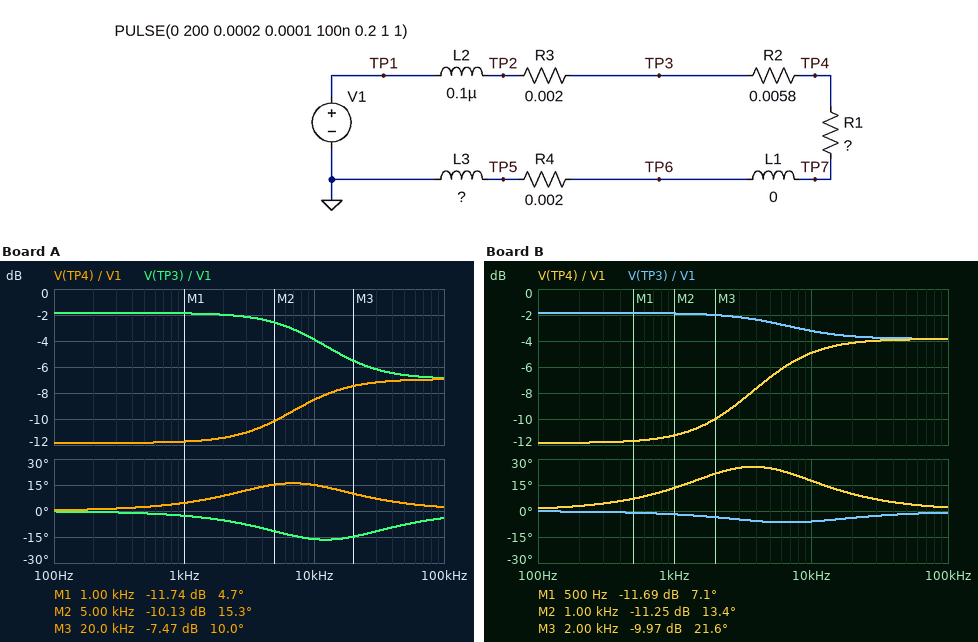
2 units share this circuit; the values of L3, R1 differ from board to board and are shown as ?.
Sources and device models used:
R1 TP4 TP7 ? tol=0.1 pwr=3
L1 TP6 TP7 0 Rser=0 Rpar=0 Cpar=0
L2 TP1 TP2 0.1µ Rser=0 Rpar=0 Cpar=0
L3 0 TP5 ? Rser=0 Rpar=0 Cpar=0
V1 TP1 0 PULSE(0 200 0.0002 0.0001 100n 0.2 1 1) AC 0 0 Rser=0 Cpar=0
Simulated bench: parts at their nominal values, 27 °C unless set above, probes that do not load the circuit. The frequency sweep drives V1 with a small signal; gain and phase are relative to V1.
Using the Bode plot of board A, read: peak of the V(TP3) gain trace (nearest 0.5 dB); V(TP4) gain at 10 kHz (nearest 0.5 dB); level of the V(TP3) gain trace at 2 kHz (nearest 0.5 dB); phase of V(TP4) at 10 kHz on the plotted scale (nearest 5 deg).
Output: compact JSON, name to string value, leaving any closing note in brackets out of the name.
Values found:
{"peak of the V(TP3) gain trace": "-2.0 dB", "V(TP4) gain at 10 kHz": "-8.5 dB", "level of the V(TP3) gain trace at 2 kHz": "-2.0 dB", "phase of V(TP4) at 10 kHz on the plotted scale": "15 deg"}
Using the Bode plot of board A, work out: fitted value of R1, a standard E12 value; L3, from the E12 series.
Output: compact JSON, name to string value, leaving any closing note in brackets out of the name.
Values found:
{"fitted value of R1, a standard E12 value": "680 µΩ", "L3, from the E12 series": "82 nH"}
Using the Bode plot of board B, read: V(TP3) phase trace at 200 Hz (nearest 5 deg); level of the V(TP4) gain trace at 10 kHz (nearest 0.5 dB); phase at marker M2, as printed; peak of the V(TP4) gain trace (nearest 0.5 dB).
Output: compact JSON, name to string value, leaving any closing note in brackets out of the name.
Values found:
{"V(TP3) phase trace at 200 Hz": "0 deg", "level of the V(TP4) gain trace at 10 kHz": "-5.0 dB", "phase at marker M2, as printed": "13.4 deg", "peak of the V(TP4) gain trace": "-4.0 dB"}
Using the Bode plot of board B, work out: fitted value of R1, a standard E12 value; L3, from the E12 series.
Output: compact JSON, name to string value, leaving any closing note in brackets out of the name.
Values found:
{"fitted value of R1, a standard E12 value": "680 µΩ", "L3, from the E12 series": "180 nH"}
